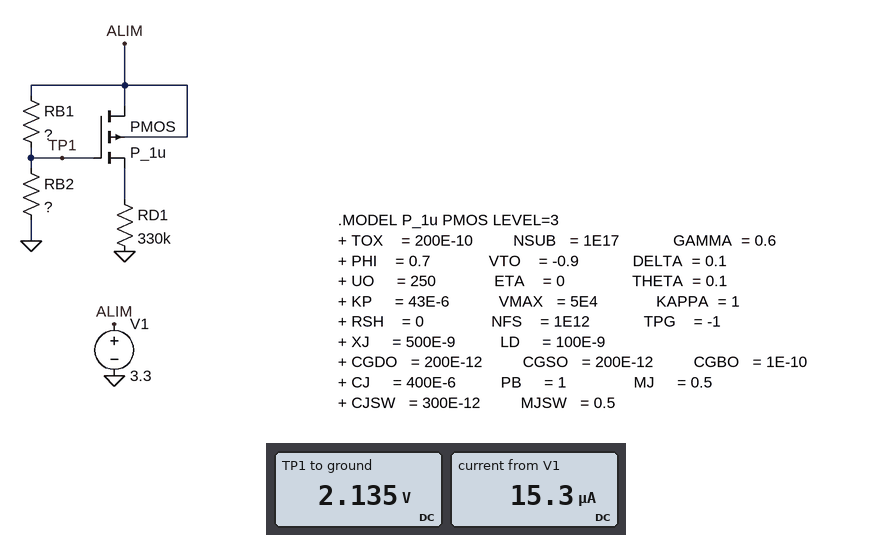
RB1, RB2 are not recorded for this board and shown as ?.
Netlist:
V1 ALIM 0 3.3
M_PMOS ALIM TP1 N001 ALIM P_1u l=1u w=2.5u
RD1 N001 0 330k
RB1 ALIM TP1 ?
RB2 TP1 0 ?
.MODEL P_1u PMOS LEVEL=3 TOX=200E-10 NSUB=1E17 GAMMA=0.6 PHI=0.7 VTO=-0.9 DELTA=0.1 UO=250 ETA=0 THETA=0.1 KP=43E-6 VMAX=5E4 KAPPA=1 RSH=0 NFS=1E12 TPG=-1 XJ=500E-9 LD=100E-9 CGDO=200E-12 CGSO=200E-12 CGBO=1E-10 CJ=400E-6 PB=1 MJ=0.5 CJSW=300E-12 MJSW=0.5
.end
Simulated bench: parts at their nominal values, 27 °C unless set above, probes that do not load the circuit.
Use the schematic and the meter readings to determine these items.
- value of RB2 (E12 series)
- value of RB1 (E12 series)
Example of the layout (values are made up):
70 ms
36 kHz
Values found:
220 kΩ
120 kΩ
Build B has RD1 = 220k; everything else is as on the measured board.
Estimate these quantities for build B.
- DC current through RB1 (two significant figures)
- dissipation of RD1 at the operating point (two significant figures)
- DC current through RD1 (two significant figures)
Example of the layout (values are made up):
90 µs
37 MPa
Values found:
9.7 µA
7.3 µW
5.8 µA
